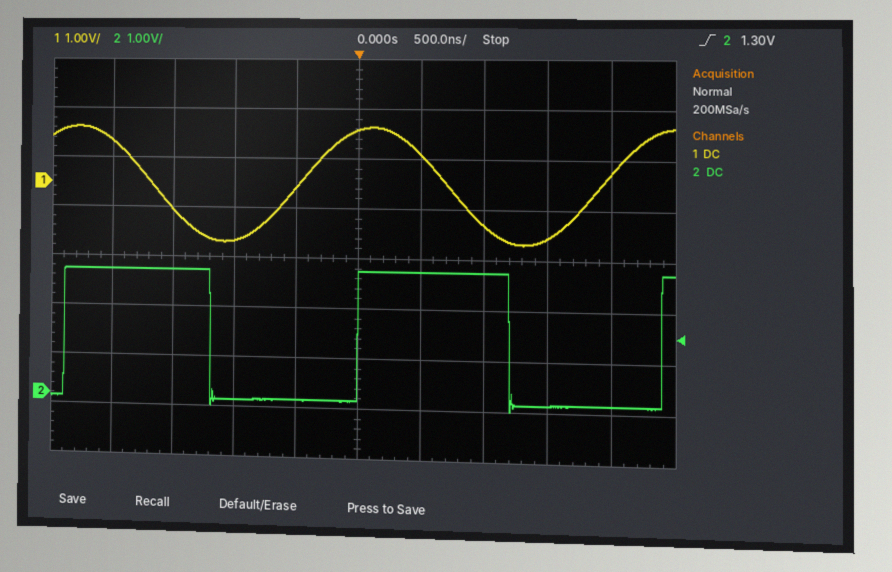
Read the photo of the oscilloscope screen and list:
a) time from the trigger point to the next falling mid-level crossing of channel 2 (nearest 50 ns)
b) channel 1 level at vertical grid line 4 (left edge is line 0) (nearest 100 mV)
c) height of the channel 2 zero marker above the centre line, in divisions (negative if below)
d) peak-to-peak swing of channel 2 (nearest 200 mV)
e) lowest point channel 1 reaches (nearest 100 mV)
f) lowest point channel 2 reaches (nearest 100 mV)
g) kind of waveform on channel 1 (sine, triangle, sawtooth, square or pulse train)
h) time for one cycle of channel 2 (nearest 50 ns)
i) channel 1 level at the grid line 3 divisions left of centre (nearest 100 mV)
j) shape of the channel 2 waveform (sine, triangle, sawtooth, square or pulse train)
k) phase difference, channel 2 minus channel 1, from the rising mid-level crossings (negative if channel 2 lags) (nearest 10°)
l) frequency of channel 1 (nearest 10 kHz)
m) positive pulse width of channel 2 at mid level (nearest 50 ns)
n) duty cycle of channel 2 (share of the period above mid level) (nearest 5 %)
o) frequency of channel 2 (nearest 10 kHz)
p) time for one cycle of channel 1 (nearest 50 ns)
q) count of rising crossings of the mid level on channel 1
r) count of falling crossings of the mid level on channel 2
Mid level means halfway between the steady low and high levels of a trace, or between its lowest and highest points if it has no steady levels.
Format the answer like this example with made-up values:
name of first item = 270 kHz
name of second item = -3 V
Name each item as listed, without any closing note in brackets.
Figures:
time from the trigger point to the next falling mid-level crossing of channel 2 = 1.20 µs
channel 1 level at vertical grid line 4 (left edge is line 0) = -100 mV
height of the channel 2 zero marker above the centre line, in divisions = -2.8 div
peak-to-peak swing of channel 2 = 2.8 V
lowest point channel 1 reaches = -1.2 V
lowest point channel 2 reaches = -200 mV
kind of waveform on channel 1 = sine
time for one cycle of channel 2 = 2.40 µs
channel 1 level at the grid line 3 divisions left of centre = -500 mV
shape of the channel 2 waveform = square
phase difference, channel 2 minus channel 1, from the rising mid-level crossings (negative if channel 2 lags) = -70°
frequency of channel 1 = 420 kHz
positive pulse width of channel 2 at mid level = 1.20 µs
duty cycle of channel 2 (share of the period above mid level) = 50 %
frequency of channel 2 = 420 kHz
time for one cycle of channel 1 = 2.40 µs
count of rising crossings of the mid level on channel 1 = 2
count of falling crossings of the mid level on channel 2 = 2
